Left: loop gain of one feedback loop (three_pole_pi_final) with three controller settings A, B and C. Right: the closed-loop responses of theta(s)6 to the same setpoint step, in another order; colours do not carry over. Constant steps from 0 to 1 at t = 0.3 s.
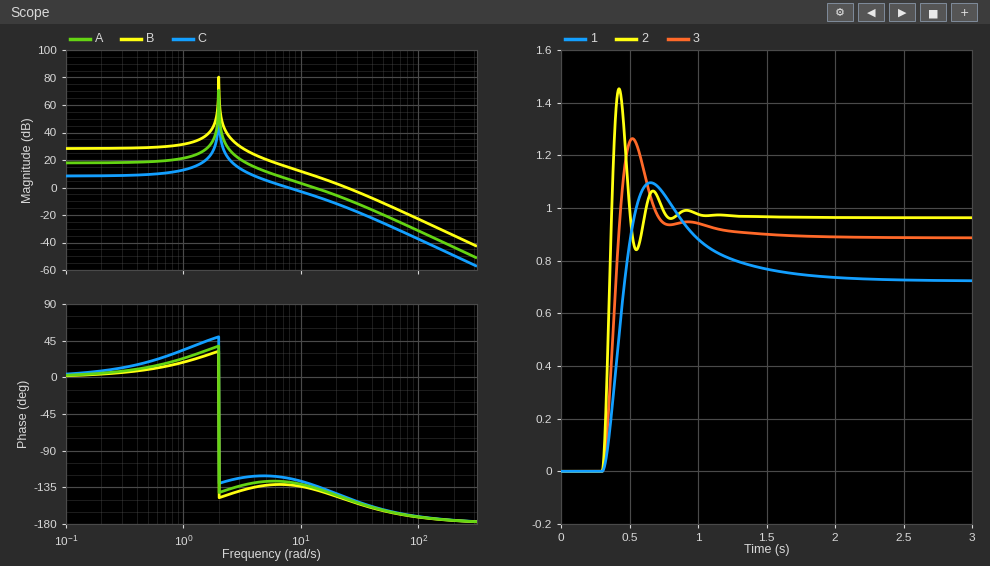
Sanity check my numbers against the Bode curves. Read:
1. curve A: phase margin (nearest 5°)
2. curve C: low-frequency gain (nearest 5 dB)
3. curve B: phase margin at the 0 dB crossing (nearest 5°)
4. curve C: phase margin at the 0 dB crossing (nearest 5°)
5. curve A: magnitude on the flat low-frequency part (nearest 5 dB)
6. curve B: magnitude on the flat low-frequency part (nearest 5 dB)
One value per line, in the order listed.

45°
10 dB
30°
55°
20 dB
30 dB
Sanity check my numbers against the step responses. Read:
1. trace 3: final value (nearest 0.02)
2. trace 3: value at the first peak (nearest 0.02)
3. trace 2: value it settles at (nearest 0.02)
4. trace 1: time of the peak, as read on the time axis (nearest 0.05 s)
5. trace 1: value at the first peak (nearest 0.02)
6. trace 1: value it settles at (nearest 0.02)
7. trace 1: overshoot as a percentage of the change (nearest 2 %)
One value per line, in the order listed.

0.88
1.26
0.96
0.65 s
1.10
0.72
52 %
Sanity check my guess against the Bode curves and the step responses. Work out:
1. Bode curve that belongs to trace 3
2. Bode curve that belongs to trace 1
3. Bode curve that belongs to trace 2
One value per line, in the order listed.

A
C
B
